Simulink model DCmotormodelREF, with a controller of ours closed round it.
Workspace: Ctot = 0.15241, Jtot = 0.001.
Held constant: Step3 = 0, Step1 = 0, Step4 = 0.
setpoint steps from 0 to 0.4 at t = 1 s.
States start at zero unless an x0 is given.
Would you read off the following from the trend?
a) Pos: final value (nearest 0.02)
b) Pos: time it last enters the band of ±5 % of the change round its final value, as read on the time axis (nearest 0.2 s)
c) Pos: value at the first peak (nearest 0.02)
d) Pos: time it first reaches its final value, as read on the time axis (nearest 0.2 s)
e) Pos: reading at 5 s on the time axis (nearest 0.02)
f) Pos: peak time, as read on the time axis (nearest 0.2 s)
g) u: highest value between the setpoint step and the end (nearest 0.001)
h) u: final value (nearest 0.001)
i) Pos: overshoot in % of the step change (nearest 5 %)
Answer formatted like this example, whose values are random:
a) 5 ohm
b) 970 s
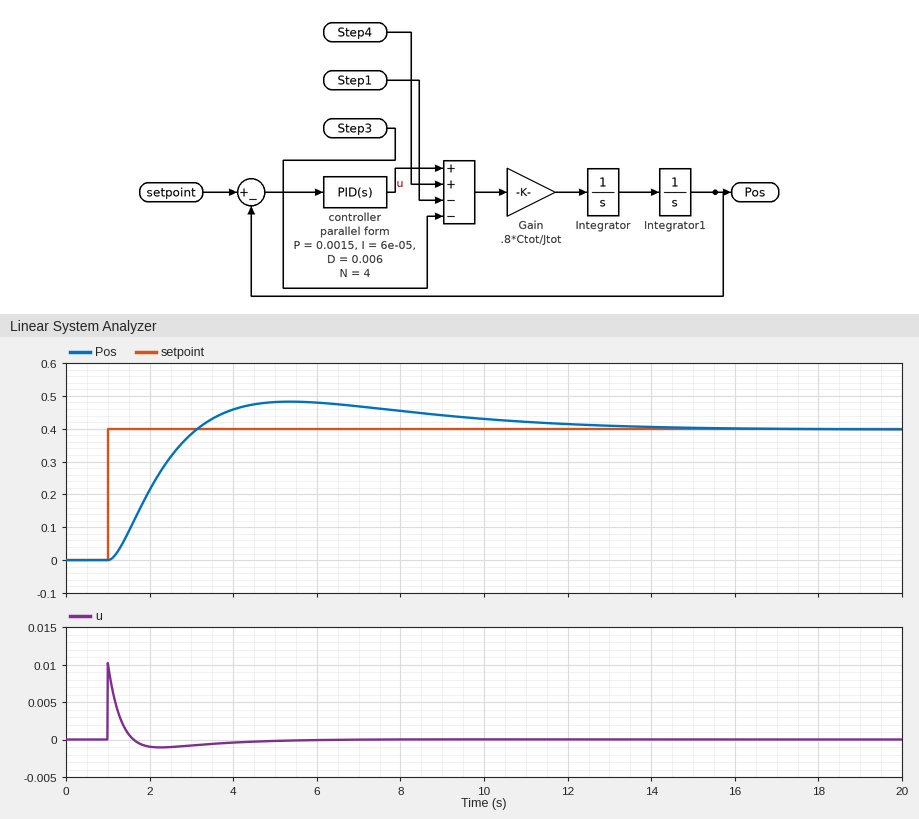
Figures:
a) 0.40
b) 11.2 s
c) 0.48
d) 3.2 s
e) 0.48
f) 5.4 s
g) 0.010
h) 0.000
i) 20 %
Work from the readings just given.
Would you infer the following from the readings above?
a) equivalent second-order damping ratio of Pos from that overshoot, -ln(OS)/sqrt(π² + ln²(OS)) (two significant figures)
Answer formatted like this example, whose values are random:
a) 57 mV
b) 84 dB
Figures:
a) 0.46
